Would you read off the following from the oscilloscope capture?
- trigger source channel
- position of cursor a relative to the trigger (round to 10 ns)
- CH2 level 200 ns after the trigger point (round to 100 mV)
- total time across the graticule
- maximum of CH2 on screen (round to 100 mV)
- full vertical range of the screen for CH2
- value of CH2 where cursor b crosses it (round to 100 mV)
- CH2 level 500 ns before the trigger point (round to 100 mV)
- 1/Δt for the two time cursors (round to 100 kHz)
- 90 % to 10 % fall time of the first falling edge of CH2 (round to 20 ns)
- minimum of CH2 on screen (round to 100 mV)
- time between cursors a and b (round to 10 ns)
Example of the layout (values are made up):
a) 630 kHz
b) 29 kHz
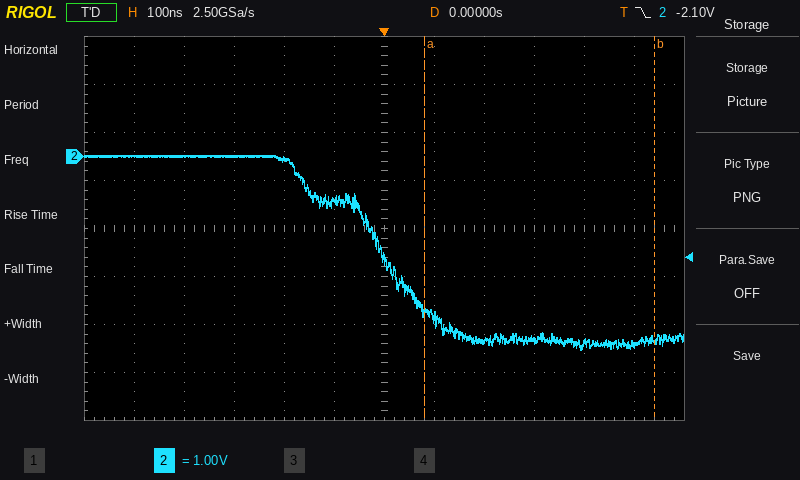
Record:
a) CH2
b) +80 ns
c) -3.8 V
d) 1.2 µs
e) 0.0 V
f) 8 V
g) -3.8 V
h) 0.0 V
i) 2.2 MHz
j) 280 ns
k) -4.0 V
l) 460 ns
